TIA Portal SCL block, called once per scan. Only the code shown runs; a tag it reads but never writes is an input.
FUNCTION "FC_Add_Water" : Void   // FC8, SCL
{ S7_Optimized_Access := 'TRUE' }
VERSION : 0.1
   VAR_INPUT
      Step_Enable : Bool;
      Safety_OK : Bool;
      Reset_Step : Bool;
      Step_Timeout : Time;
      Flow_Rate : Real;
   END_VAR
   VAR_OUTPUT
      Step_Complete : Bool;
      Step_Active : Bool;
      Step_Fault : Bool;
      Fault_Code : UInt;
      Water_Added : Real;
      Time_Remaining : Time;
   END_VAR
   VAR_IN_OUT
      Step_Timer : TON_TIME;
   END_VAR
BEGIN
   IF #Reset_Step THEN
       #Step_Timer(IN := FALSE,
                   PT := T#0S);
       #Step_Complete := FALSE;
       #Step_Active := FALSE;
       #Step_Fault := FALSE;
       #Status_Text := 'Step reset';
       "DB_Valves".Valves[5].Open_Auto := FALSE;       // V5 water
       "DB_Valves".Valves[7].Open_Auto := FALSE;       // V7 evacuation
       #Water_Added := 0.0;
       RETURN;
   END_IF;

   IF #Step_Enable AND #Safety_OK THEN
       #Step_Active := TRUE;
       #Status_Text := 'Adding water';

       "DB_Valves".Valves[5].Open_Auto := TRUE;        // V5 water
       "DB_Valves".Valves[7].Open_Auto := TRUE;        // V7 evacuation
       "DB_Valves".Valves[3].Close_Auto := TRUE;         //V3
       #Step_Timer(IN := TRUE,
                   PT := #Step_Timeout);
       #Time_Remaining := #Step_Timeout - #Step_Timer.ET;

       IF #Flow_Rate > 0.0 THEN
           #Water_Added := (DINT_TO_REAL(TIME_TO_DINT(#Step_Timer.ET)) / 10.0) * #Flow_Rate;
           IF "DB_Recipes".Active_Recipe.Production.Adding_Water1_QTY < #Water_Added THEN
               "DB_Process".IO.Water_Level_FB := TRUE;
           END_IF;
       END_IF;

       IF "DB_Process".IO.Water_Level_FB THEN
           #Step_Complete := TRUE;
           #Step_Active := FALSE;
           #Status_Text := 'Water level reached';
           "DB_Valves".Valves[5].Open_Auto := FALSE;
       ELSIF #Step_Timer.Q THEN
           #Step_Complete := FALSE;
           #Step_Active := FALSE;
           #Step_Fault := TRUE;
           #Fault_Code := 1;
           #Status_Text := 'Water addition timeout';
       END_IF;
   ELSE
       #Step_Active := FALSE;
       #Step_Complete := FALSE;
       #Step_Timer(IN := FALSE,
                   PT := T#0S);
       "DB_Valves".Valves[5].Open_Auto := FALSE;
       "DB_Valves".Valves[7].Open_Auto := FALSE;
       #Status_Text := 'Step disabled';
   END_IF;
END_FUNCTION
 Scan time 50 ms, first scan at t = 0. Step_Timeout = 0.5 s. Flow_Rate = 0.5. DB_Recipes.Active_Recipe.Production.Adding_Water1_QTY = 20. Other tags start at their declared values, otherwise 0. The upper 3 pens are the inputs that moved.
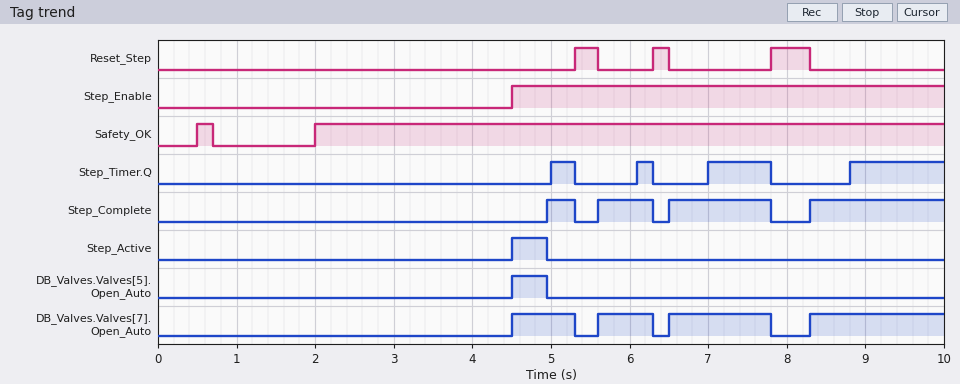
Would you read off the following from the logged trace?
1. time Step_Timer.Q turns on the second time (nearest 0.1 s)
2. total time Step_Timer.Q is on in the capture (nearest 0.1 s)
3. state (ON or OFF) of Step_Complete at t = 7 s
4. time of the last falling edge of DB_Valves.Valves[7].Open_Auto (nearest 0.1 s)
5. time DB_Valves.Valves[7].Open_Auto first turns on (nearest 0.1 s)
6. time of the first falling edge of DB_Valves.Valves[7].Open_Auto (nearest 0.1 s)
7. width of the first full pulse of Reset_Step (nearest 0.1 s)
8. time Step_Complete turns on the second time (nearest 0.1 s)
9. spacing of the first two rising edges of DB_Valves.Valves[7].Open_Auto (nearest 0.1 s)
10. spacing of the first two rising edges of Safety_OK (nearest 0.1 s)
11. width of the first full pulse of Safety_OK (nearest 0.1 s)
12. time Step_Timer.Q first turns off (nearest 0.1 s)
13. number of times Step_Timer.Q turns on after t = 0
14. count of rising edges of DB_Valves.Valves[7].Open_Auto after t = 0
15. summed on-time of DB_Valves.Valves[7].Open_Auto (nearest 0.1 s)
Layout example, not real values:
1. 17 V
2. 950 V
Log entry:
1. 6.1 s
2. 2.5 s
3. ON
4. 7.8 s
5. 4.5 s
6. 5.3 s
7. 0.3 s
8. 5.6 s
9. 1.1 s
10. 1.5 s
11. 0.2 s
12. 5.3 s
13. 4
14. 4
15. 4.5 s
